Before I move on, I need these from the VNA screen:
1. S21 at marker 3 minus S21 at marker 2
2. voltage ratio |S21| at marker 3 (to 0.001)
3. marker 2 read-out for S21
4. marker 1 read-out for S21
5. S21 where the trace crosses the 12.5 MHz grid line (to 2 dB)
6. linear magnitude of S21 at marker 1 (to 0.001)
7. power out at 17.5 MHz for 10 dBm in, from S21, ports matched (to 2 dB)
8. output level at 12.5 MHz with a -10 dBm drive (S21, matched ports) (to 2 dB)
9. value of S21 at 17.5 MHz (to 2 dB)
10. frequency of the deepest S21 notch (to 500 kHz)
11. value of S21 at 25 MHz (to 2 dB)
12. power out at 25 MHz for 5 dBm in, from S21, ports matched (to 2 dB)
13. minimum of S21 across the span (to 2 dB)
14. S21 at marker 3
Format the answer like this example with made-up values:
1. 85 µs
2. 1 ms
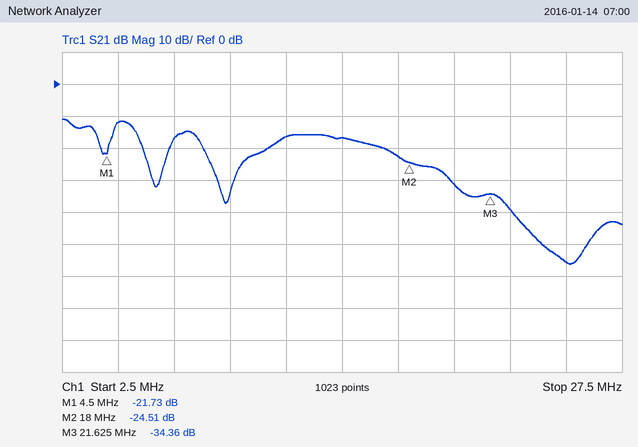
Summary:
1. -9.85 dB
2. 0.019
3. -24.51 dB
4. -21.73 dB
5. -16 dB
6. 0.082
7. -12 dBm
8. -26 dBm
9. -22 dB
10. 25.0 MHz
11. -56 dB
12. -50 dBm
13. -56 dB
14. -34.36 dB
